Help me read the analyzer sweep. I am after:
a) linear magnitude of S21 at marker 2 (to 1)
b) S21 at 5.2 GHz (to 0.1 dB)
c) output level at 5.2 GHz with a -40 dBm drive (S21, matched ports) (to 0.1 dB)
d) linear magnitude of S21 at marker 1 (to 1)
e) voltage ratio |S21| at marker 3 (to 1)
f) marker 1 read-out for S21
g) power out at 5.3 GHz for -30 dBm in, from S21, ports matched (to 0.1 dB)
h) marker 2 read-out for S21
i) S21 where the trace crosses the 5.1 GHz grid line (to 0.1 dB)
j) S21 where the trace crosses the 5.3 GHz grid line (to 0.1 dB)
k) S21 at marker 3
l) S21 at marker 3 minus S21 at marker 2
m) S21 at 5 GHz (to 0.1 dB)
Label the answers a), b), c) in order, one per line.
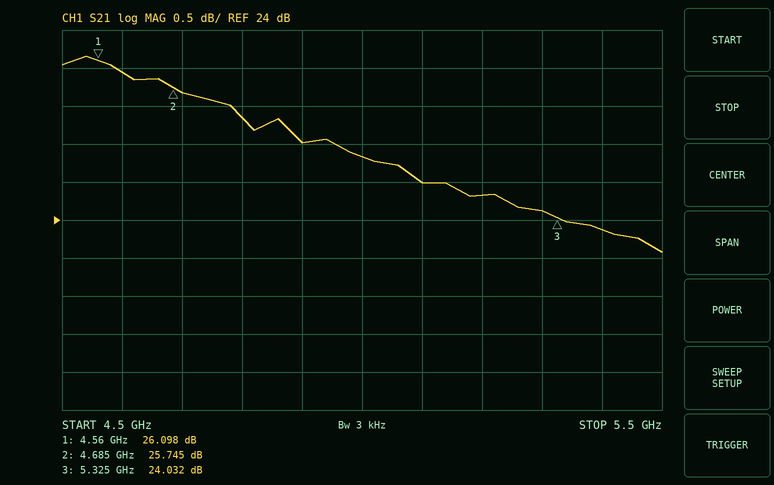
a) 19
b) 24.3 dB
c) -15.7 dBm
d) 20
e) 16
f) 26.098 dB
g) -5.9 dBm
h) 25.745 dB
i) 24.5 dB
j) 24.1 dB
k) 24.032 dB
l) -1.713 dB
m) 24.8 dB
